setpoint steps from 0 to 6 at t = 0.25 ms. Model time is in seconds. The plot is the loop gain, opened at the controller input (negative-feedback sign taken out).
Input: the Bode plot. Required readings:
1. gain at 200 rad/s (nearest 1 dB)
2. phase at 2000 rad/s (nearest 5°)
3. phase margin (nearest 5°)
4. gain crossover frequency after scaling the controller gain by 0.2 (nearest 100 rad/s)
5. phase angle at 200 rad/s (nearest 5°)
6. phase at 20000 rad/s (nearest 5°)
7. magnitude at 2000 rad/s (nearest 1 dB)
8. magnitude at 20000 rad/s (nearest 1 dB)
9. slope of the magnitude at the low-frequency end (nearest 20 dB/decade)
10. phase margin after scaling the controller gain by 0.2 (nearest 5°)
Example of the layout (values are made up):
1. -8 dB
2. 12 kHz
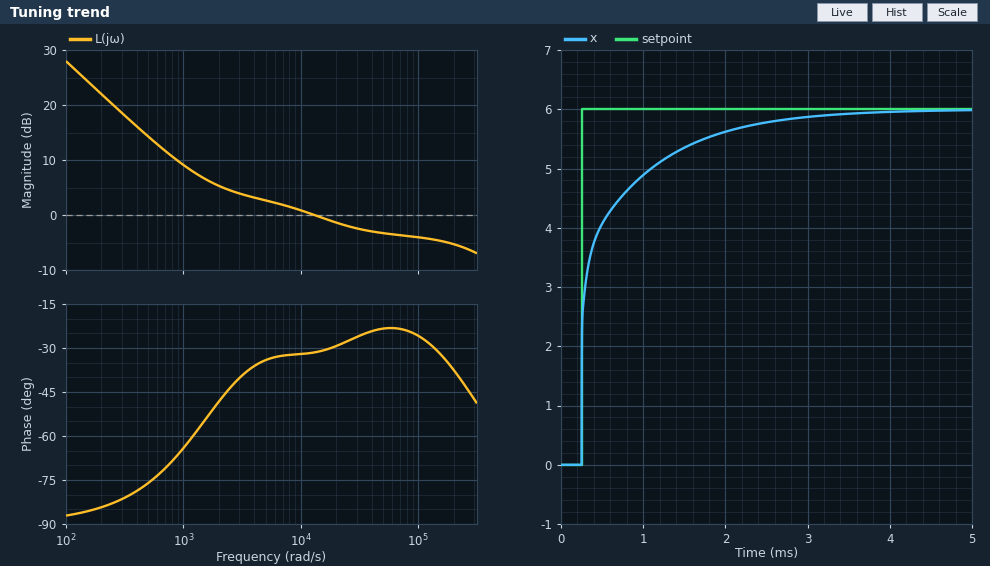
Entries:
1. 22 dB
2. -50°
3. 150°
4. 500 rad/s
5. -85°
6. -30°
7. 5 dB
8. -1 dB
9. -20 dB/decade
10. 105°
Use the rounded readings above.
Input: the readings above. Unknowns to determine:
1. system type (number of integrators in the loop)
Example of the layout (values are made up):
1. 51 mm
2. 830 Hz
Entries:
1. 1
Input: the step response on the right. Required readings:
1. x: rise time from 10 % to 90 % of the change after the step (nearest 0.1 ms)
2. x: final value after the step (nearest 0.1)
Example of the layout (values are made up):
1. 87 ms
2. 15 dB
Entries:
1. 1.3 ms
2. 6.0
